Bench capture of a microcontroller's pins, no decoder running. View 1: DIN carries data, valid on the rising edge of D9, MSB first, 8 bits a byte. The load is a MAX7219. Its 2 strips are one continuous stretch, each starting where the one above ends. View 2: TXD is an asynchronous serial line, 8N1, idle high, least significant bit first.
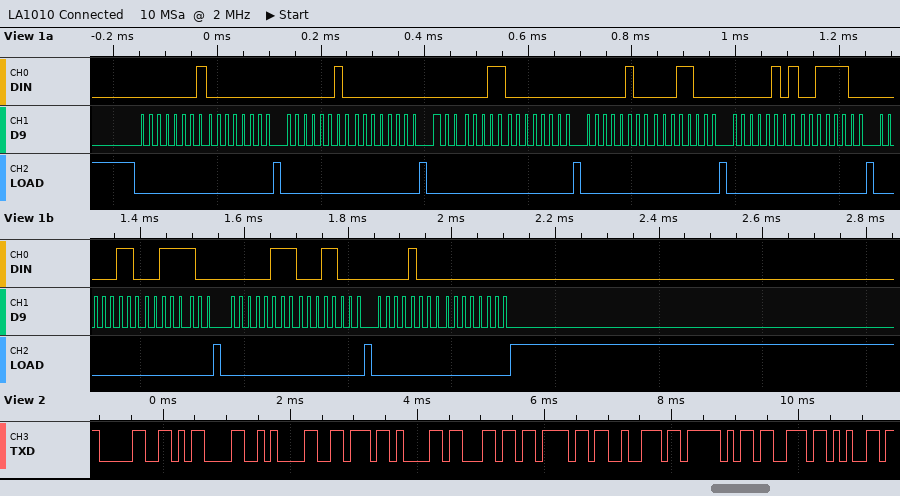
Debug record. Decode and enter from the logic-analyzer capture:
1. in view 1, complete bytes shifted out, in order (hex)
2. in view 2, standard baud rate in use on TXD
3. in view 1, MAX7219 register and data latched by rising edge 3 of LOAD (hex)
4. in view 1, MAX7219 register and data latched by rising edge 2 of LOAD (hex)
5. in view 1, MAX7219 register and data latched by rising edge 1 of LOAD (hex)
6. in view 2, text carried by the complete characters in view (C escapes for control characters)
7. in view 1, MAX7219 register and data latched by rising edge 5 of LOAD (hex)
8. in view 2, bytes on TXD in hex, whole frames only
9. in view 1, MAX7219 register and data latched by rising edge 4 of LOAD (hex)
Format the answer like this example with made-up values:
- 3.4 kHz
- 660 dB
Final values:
- 0x01 0x00 0x02 0x00 0x03 0x00 0x04 0x18 0x05 0x3C 0x06 0x3C 0x07 0x18 0x08 0x00
- 9600 baud
- register 0x3, data 0x00
- register 0x2, data 0x00
- register 0x1, data 0x00
- "0\r\nvalor_se"
- register 0x5, data 0x3C
- 30 0D 0A 76 61 6C 6F 72 5F 73 65
- register 0x4, data 0x18
